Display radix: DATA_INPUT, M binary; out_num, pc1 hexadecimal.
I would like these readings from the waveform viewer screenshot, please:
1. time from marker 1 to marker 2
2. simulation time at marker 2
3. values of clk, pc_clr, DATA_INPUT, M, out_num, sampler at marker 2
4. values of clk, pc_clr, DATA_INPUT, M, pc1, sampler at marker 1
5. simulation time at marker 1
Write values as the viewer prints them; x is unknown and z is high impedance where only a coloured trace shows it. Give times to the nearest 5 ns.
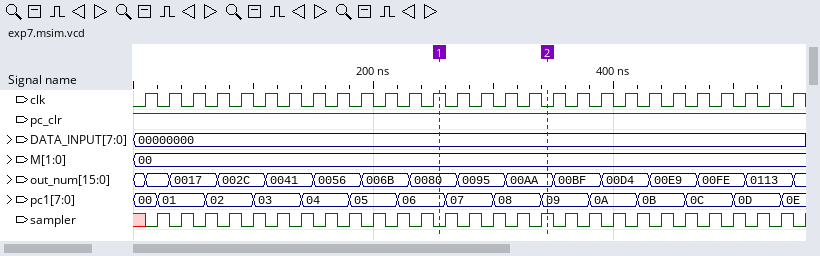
90 ns
345 ns
clk=0, pc_clr=1, DATA_INPUT=00000000, M=00, out_num=00AA, sampler=1
clk=1, pc_clr=1, DATA_INPUT=00000000, M=00, pc1=06, sampler=0
255 ns
